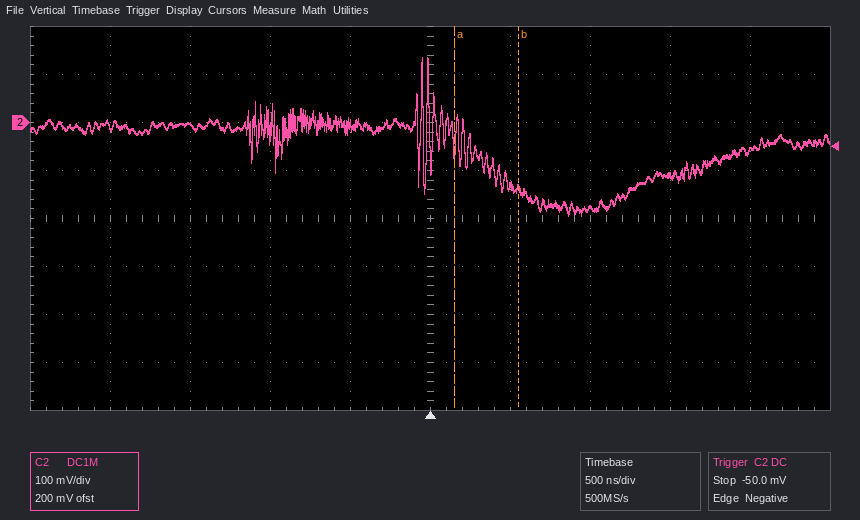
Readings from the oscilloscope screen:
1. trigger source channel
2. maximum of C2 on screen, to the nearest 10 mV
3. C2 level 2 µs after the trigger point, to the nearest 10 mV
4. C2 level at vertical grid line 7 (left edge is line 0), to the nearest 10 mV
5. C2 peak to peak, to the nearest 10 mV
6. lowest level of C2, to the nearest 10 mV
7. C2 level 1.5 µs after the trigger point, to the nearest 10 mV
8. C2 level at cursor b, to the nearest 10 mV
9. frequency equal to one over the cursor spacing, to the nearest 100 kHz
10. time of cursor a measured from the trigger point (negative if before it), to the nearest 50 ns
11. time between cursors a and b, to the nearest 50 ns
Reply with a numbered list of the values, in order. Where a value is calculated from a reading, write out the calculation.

1. C2
2. 140 mV
3. -60 mV
4. -180 mV
5. 140 mV − (-190 mV) = 330 mV
6. -190 mV
7. -110 mV
8. -140 mV
9. 1 / 400 ns ≈ 2.5 MHz
10. +150 ns
11. 400 ns
